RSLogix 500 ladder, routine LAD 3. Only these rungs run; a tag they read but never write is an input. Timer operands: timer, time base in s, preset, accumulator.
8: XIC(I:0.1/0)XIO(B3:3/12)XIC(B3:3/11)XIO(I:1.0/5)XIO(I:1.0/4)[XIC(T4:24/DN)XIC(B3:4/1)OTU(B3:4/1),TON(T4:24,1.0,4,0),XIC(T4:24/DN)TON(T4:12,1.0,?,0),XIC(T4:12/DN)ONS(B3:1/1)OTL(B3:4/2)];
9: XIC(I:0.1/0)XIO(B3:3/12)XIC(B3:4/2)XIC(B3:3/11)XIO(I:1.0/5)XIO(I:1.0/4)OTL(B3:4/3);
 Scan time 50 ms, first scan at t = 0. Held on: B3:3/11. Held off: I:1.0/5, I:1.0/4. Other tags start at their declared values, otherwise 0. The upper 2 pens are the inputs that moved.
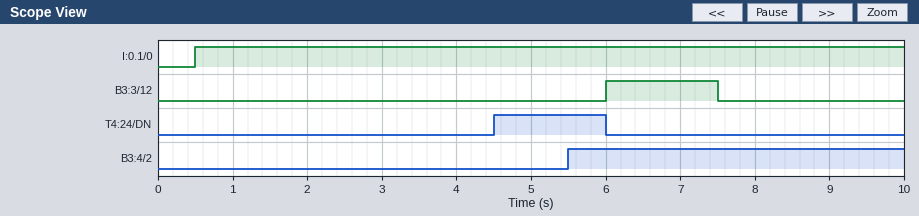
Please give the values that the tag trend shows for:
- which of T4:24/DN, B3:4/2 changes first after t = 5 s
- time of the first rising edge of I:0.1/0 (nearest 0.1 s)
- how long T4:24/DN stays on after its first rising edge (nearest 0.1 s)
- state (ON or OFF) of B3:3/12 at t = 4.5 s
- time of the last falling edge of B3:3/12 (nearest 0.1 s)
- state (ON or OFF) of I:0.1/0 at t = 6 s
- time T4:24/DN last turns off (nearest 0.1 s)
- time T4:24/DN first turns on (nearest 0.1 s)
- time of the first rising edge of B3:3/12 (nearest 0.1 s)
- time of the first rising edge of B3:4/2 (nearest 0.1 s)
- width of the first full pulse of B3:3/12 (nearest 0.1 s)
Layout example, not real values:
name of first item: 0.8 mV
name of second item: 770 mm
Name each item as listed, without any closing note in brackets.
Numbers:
which of T4:24/DN, B3:4/2 changes first after t = 5 s: B3:4/2
time of the first rising edge of I:0.1/0: 0.5 s
how long T4:24/DN stays on after its first rising edge: 1.5 s
state (ON or OFF) of B3:3/12 at t = 4.5 s: OFF
time of the last falling edge of B3:3/12: 7.5 s
state (ON or OFF) of I:0.1/0 at t = 6 s: ON
time T4:24/DN last turns off: 6.0 s
time T4:24/DN first turns on: 4.5 s
time of the first rising edge of B3:3/12: 6.0 s
time of the first rising edge of B3:4/2: 5.5 s
width of the first full pulse of B3:3/12: 1.5 s
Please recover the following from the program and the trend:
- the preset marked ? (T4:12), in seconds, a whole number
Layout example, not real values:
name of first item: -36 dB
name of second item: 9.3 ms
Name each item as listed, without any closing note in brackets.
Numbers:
the preset marked ? (T4:12), in seconds, a whole number: 1 s
